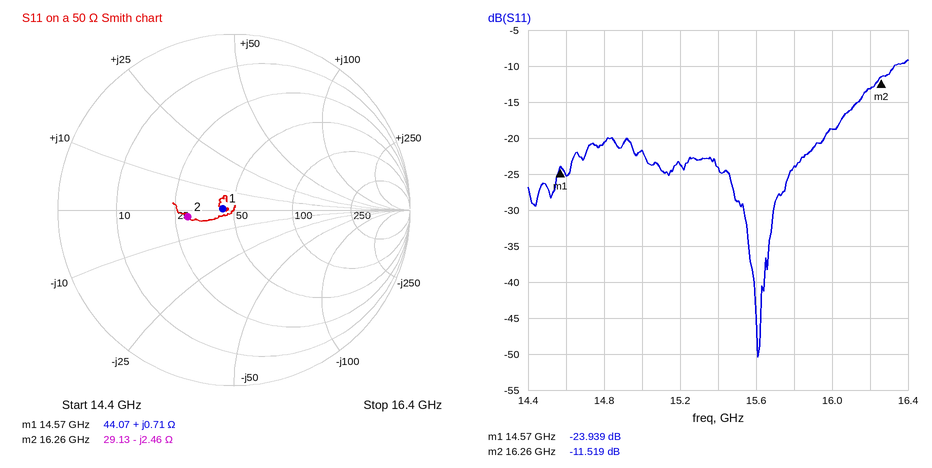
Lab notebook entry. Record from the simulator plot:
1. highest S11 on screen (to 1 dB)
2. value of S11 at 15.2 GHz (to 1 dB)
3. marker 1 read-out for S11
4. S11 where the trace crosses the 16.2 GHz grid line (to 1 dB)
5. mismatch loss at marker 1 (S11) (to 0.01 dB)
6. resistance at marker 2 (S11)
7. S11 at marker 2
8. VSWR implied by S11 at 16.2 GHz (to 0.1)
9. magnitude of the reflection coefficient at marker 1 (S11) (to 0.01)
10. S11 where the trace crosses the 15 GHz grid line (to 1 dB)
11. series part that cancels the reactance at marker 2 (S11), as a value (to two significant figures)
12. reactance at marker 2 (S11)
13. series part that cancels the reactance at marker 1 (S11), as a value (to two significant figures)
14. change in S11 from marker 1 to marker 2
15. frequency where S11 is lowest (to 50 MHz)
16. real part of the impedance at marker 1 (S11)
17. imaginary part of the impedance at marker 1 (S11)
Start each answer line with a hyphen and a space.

- -9 dB
- -24 dB
- -23.939 dB
- -13 dB
- 0.02 dB
- 29.13 Ω
- -11.519 dB
- 1.6
- 0.06
- -22 dB
- 24 pH
- -2.46 Ω
- 15 pF
- 12.420 dB
- 15.60 GHz
- 44.07 Ω
- +0.71 Ω
